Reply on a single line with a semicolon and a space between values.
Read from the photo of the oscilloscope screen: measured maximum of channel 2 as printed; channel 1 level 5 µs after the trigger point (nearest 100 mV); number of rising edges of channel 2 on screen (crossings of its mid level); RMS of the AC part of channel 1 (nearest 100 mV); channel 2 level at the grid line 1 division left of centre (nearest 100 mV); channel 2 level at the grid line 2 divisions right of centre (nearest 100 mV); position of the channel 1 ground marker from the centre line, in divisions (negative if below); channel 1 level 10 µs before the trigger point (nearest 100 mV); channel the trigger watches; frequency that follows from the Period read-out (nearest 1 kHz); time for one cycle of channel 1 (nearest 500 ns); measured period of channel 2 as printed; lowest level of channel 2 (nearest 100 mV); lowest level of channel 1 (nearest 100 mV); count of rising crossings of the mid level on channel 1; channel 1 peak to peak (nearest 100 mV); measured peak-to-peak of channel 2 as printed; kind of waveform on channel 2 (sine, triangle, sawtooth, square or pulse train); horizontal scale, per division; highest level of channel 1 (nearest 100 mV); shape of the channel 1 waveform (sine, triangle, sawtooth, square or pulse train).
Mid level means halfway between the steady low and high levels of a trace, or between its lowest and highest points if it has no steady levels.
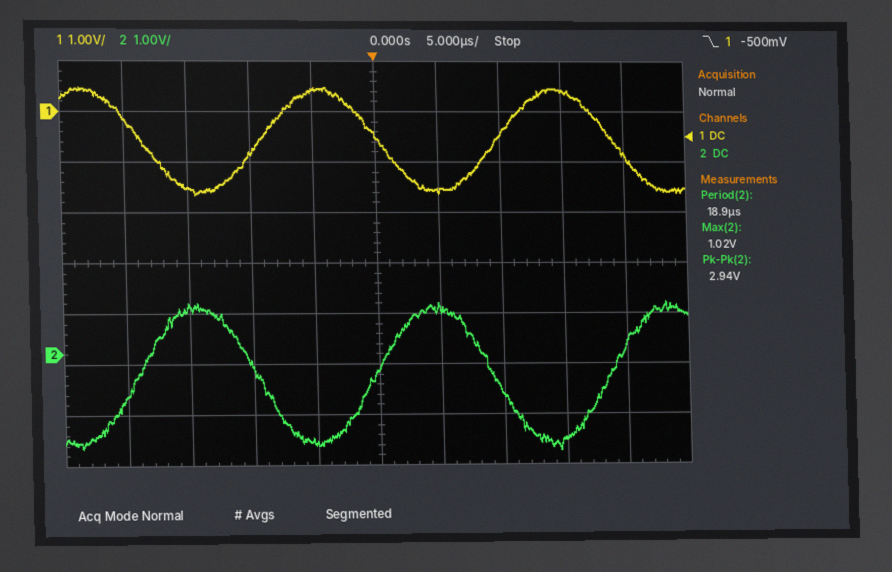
1.02 V; -1.6 V; 3; 700 mV; -1.8 V; -800 mV; +3.0 div; -800 mV; channel 1; 53 kHz; 19.0 µs; 18.9 µs; -1.9 V; -1.6 V; 2; 2.1 V; 2.94 V; sine; 5 µs; 500 mV; sine
